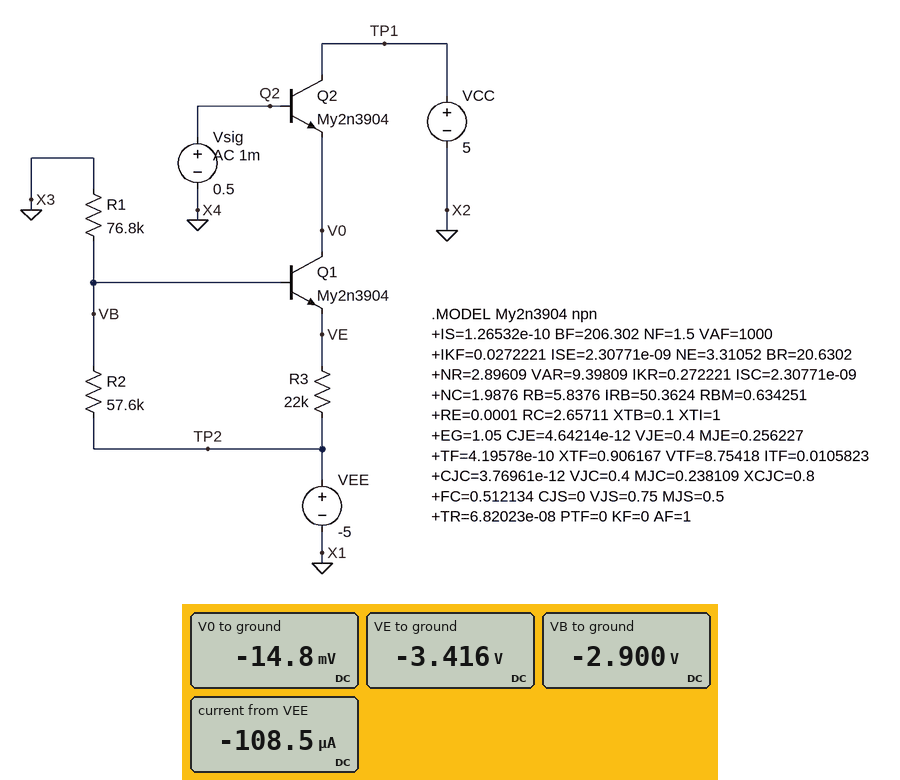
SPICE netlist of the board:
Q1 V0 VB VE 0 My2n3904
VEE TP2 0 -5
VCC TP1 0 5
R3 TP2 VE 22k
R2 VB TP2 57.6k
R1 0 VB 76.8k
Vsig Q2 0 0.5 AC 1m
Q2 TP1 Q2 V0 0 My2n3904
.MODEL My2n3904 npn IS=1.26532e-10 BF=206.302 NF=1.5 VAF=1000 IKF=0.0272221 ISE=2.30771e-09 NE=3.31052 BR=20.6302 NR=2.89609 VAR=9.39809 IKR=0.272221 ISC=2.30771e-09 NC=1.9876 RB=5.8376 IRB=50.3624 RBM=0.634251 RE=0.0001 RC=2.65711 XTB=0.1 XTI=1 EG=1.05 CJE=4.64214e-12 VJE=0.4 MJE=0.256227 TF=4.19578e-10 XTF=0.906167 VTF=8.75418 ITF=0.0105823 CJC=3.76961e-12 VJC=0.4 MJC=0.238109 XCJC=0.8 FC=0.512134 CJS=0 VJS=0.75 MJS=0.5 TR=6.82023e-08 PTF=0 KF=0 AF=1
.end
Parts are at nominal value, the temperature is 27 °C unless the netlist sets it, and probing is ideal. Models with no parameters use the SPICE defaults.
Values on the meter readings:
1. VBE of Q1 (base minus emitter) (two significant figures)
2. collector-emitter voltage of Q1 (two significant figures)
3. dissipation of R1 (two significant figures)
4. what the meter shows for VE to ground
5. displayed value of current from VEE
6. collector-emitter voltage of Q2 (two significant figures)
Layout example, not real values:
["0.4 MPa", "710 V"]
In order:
["520 mV", "3.4 V", "110 µW", "-3.416 V", "-108.5 µA", "5.0 V"]
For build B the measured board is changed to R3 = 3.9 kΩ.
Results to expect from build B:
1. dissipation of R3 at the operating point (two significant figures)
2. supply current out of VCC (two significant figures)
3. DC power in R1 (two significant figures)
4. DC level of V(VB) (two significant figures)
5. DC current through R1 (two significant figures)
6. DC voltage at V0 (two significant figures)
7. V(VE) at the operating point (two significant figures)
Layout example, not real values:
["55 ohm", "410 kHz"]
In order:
["530 µW", "360 µA", "120 µW", "-3.0 V", "39 µA", "-79 mV", "-3.6 V"]
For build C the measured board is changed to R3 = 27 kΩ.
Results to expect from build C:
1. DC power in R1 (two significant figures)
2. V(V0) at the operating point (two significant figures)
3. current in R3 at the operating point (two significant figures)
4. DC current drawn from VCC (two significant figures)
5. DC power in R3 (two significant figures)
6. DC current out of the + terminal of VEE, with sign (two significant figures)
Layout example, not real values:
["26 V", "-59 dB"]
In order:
["110 µW", "-7.0 mV", "59 µA", "57 µA", "94 µW", "-96 µA"]
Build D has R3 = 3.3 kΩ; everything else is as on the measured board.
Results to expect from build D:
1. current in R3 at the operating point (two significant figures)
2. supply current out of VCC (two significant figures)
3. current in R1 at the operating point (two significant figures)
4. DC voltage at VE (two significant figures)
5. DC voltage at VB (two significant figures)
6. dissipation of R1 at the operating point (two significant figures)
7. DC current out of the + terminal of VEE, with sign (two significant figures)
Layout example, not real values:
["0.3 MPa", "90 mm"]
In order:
["430 µA", "420 µA", "39 µA", "-3.6 V", "-3.0 V", "120 µW", "-460 µA"]
